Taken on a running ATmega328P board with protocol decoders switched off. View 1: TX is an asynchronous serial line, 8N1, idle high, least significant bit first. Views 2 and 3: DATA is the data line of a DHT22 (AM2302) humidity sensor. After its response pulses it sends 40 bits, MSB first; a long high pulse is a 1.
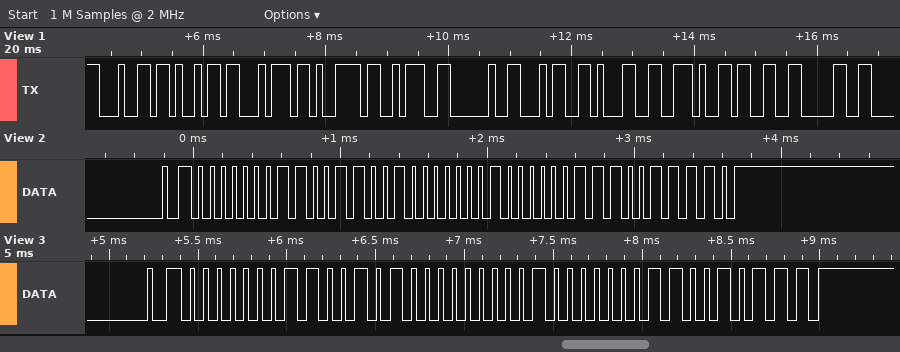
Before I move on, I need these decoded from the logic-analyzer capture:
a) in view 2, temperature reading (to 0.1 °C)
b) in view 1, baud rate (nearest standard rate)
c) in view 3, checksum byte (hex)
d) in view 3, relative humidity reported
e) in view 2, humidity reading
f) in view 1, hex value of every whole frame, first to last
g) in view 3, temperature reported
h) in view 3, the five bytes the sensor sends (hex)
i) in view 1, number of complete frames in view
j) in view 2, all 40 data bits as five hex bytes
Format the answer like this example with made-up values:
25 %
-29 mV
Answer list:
25.9 °C
9600 baud
0x97
40.4 %
40.9 %
64 69 74 79 3A 20 34 31 2E 33 30
25.7 °C
01 94 01 01 97
11
01 99 01 03 9E
